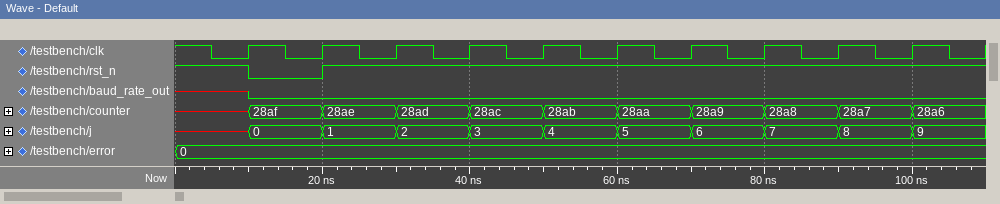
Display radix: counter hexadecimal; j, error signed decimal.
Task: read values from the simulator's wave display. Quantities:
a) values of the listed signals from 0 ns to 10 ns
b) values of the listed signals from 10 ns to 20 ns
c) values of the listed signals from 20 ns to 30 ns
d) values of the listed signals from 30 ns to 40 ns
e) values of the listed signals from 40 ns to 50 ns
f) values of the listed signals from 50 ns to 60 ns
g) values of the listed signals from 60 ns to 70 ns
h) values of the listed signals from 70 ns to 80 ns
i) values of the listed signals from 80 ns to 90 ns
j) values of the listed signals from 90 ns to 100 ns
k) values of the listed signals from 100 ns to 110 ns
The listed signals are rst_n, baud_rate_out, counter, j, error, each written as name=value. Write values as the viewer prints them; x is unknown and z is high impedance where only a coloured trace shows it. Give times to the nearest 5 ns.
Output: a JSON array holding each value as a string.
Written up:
["rst_n=1, baud_rate_out=x, counter=x, j=x, error=0", "rst_n=0, baud_rate_out=0, counter=28af, j=0, error=0", "rst_n=1, baud_rate_out=0, counter=28ae, j=1, error=0", "rst_n=1, baud_rate_out=0, counter=28ad, j=2, error=0", "rst_n=1, baud_rate_out=0, counter=28ac, j=3, error=0", "rst_n=1, baud_rate_out=0, counter=28ab, j=4, error=0", "rst_n=1, baud_rate_out=0, counter=28aa, j=5, error=0", "rst_n=1, baud_rate_out=0, counter=28a9, j=6, error=0", "rst_n=1, baud_rate_out=0, counter=28a8, j=7, error=0", "rst_n=1, baud_rate_out=0, counter=28a7, j=8, error=0", "rst_n=1, baud_rate_out=0, counter=28a6, j=9, error=0"]
